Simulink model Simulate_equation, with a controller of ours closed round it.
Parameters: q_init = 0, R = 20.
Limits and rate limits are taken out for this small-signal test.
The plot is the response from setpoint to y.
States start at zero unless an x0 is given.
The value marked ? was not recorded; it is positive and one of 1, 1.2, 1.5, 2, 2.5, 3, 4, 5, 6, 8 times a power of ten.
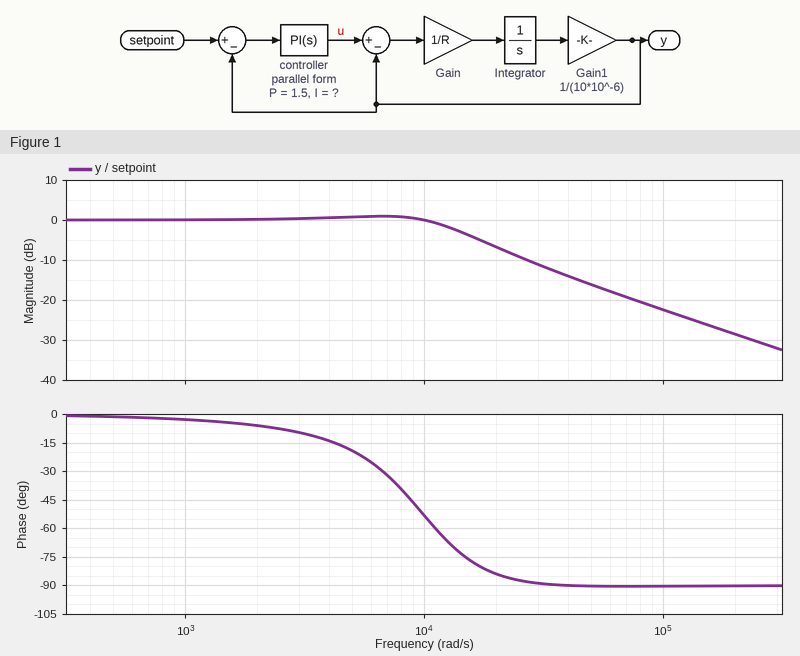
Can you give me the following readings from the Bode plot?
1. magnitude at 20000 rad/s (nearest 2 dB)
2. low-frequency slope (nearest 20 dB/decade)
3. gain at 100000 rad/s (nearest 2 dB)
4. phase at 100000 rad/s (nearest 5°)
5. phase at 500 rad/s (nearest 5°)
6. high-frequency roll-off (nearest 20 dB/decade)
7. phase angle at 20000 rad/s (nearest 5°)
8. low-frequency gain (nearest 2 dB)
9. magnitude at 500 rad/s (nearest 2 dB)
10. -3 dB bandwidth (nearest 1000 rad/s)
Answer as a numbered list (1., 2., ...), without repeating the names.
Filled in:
1. -6 dB
2. 0 dB/decade
3. -22 dB
4. -90°
5. 0°
6. -20 dB/decade
7. -85°
8. 0 dB
9. 0 dB
10. 14000 rad/s
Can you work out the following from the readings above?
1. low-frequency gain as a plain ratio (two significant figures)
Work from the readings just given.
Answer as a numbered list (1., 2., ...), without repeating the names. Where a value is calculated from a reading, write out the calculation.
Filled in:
1. 10^(0 / 20) = 1.0
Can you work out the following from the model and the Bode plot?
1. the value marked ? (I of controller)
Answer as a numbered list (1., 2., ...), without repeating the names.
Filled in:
1. 20000
